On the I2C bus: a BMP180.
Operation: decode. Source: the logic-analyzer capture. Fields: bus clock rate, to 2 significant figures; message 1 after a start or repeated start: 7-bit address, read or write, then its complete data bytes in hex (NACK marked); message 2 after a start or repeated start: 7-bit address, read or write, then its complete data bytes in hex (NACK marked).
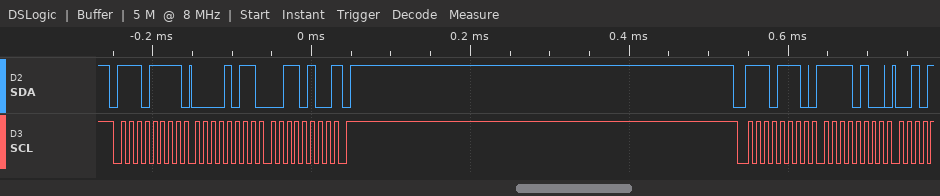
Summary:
100 kHz
0x77 read: 0B 34 NACK
0x77 write: F4
